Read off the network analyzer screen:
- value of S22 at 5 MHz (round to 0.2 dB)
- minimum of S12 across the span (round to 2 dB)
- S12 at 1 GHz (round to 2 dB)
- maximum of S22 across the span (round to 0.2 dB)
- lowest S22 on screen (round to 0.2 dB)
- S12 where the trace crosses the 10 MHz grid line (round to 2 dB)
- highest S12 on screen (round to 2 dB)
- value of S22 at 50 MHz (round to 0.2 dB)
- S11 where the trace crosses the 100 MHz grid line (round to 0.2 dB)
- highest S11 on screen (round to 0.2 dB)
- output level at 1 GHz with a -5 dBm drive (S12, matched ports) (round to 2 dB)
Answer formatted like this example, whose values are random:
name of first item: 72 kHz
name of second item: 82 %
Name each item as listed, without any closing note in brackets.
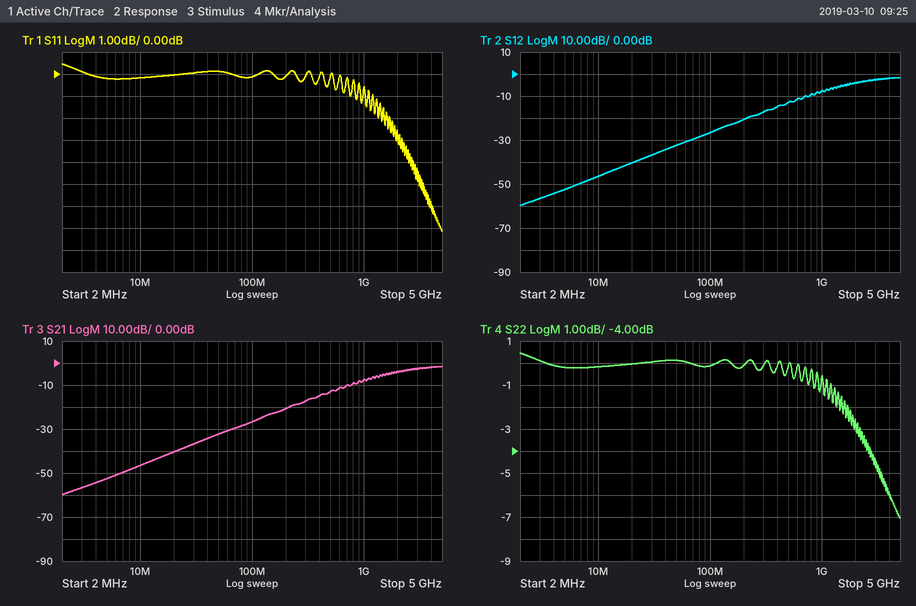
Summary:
value of S22 at 5 MHz: -0.2 dB
minimum of S12 across the span: -60 dB
S12 at 1 GHz: -8 dB
maximum of S22 across the span: 0.4 dB
lowest S22 on screen: -7.0 dB
S12 where the trace crosses the 10 MHz grid line: -46 dB
highest S12 on screen: -2 dB
value of S22 at 50 MHz: 0.2 dB
S11 where the trace crosses the 100 MHz grid line: -0.2 dB
highest S11 on screen: 0.4 dB
output level at 1 GHz with a -5 dBm drive (S12, matched ports): -12 dBm
